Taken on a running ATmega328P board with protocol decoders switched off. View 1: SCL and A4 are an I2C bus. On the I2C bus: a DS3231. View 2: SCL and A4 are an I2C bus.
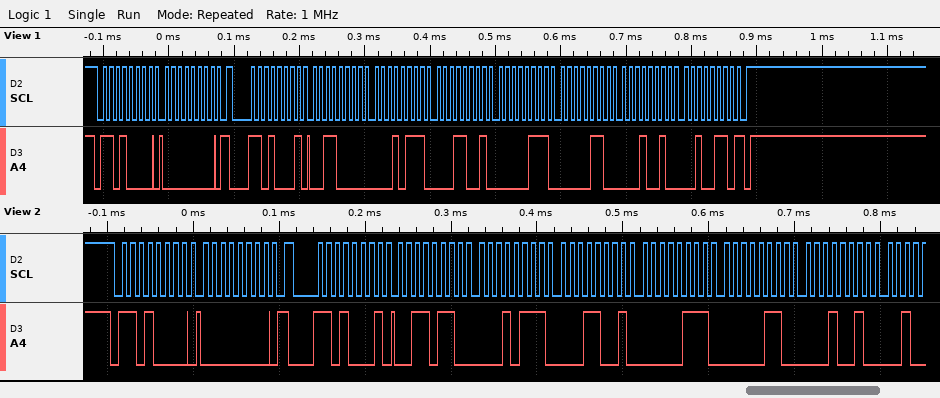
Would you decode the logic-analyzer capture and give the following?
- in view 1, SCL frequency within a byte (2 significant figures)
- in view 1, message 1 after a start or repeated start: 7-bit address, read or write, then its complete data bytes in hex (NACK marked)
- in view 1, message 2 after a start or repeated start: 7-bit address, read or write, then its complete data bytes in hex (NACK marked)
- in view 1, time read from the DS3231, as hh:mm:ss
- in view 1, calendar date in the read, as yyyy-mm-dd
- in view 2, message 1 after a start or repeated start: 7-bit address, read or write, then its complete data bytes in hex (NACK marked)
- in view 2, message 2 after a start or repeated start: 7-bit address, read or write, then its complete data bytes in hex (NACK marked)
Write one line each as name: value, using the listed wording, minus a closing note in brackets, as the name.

in view 1, SCL frequency within a byte: 100 kHz
in view 1, message 1 after a start or repeated start: 7-bit address, read or write, then its complete data bytes in hex: 0x68 write: 00
in view 1, message 2 after a start or repeated start: 7-bit address, read or write, then its complete data bytes in hex: 0x68 read: 30 17 19 07 06 12 26 NACK
in view 1, time read from the DS3231, as hh:mm:ss: 19:17:30
in view 1, calendar date in the read, as yyyy-mm-dd: 2026-12-06
in view 2, message 1 after a start or repeated start: 7-bit address, read or write, then its complete data bytes in hex: 0x68 write: 00
in view 2, message 2 after a start or repeated start: 7-bit address, read or write, then its complete data bytes in hex: 0x68 read: 36 17 19 07 06 12
